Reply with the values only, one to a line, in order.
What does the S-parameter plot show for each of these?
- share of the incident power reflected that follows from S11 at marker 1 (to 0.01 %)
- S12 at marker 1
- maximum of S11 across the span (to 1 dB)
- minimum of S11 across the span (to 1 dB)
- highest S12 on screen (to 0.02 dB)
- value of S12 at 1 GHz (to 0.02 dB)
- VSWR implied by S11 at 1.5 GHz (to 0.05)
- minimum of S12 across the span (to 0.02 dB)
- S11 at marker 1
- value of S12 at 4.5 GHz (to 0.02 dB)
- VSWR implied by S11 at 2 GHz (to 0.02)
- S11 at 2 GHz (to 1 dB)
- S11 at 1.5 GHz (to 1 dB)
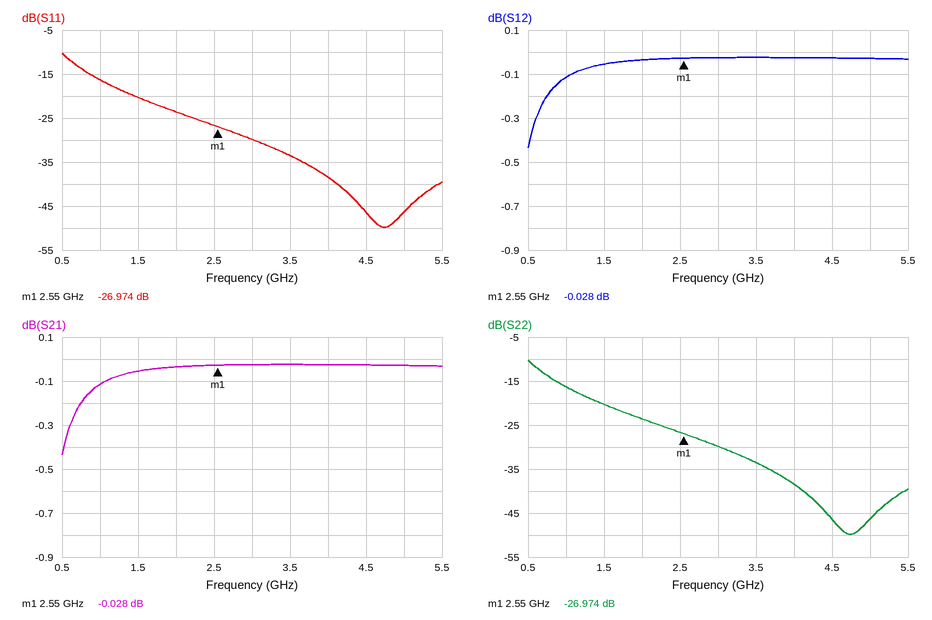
0.20 %
-0.028 dB
-10 dB
-50 dB
-0.02 dB
-0.12 dB
1.20
-0.44 dB
-26.974 dB
-0.02 dB
1.14
-24 dB
-20 dB
